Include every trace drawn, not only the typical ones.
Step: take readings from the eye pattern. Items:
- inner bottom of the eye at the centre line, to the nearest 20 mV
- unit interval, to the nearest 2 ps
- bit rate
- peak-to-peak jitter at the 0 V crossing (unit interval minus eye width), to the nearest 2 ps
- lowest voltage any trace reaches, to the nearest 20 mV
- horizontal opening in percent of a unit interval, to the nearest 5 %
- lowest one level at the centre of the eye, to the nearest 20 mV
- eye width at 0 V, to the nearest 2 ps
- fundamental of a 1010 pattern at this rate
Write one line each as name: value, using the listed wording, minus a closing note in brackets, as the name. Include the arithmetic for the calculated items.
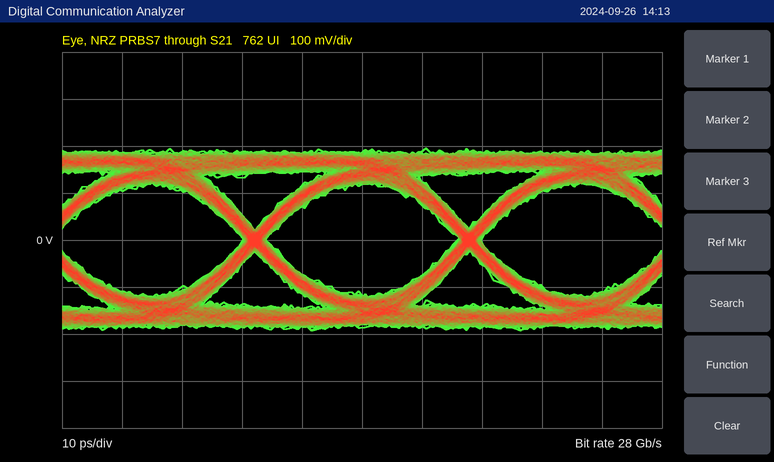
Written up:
inner bottom of the eye at the centre line, to the nearest 20 mV: -120 mV
unit interval, to the nearest 2 ps: 36 ps
bit rate: 28 Gb/s
peak-to-peak jitter at the 0 V crossing (unit interval minus eye width), to the nearest 2 ps: 4 ps
lowest voltage any trace reaches, to the nearest 20 mV: -200 mV
horizontal opening in percent of a unit interval, to the nearest 5 %: 32 ps / 36 ps ≈ 88.9 %, so 90 % to the nearest 5 %
lowest one level at the centre of the eye, to the nearest 20 mV: 120 mV
eye width at 0 V, to the nearest 2 ps: 32 ps
fundamental of a 1010 pattern at this rate: 14 GHz
